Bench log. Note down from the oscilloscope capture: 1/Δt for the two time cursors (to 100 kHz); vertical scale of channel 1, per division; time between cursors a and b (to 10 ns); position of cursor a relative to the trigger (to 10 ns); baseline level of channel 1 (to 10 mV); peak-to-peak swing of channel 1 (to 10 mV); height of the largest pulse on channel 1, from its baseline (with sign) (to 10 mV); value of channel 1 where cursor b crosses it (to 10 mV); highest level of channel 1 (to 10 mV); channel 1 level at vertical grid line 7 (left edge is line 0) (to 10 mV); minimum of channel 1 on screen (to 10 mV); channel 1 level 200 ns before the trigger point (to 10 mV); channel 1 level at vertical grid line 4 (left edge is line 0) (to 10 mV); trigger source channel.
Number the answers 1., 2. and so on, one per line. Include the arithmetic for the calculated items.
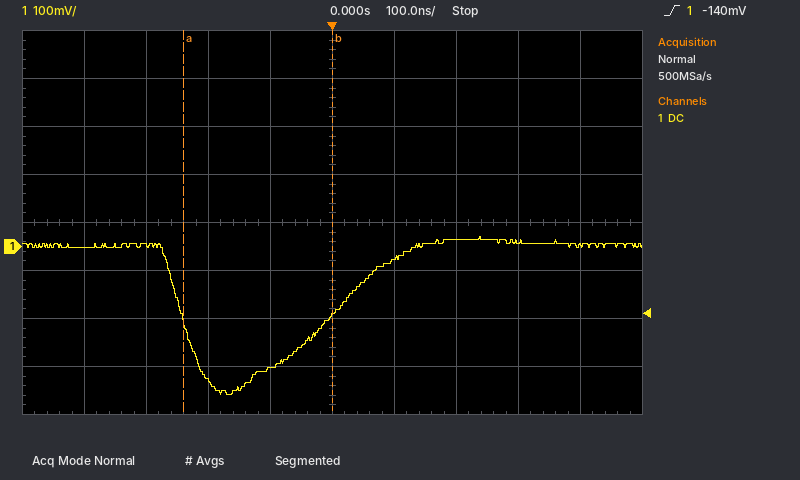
1. 1 / 240 ns ≈ 4.2 MHz
2. 100 mV
3. 240 ns
4. -240 ns
5. 0 mV
6. 20 mV − (-310 mV) = 330 mV
7. -310 mV − (0 mV) = -310 mV
8. -140 mV
9. 20 mV
10. 10 mV
11. -310 mV
12. -280 mV
13. -250 mV
14. channel 1
